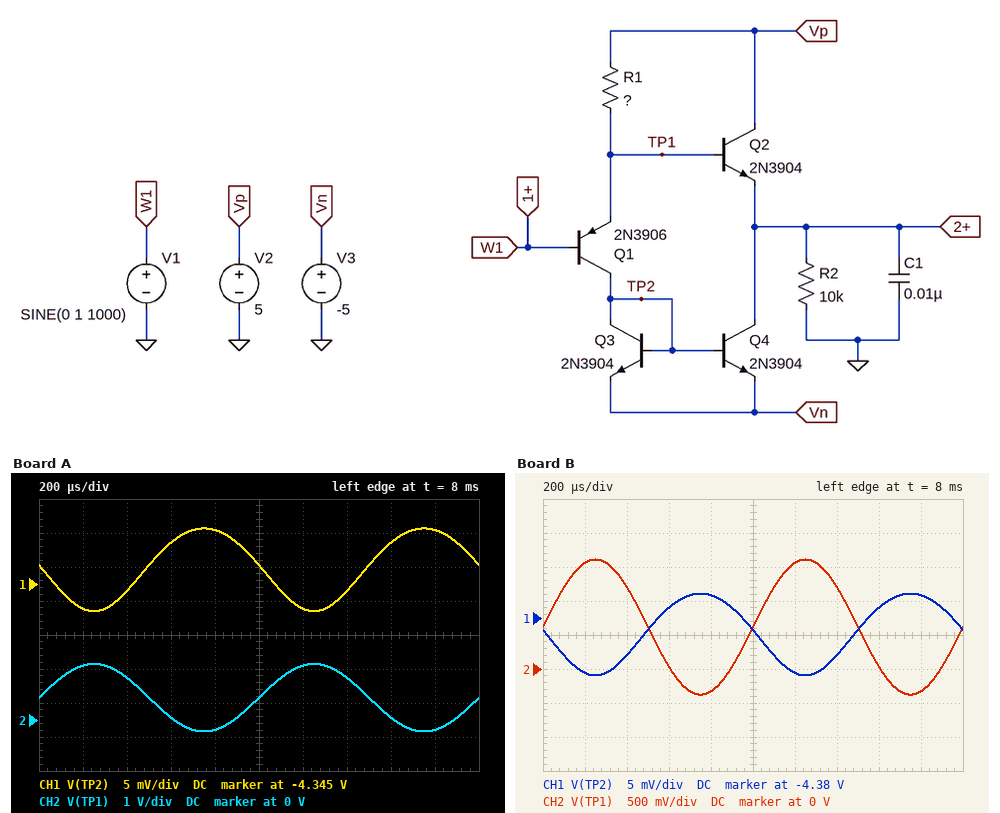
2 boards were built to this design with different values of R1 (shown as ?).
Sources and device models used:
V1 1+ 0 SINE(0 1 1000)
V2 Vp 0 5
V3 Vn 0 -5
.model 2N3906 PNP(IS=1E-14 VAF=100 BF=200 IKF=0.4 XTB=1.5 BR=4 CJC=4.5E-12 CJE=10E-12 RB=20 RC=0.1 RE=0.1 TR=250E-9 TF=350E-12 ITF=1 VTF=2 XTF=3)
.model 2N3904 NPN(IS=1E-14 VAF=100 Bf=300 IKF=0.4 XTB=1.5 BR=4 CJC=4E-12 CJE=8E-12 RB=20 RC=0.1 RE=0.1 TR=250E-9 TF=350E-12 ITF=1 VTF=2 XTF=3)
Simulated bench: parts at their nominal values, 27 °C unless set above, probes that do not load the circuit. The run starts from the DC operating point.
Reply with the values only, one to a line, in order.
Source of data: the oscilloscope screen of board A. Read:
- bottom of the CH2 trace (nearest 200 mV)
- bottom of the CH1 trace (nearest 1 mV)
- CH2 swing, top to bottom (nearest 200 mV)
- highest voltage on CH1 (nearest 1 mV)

-400 mV
-4.349 V
2.0 V
-4.337 V
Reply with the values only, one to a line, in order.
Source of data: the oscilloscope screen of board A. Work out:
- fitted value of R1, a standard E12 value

3.9 kΩ
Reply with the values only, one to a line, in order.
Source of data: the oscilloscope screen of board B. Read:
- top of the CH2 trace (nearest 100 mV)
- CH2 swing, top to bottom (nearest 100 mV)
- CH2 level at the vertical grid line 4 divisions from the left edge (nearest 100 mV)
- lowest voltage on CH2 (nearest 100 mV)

1.6 V
2.0 V
-300 mV
-400 mV
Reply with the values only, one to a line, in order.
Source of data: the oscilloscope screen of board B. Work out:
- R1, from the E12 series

18 kΩ
